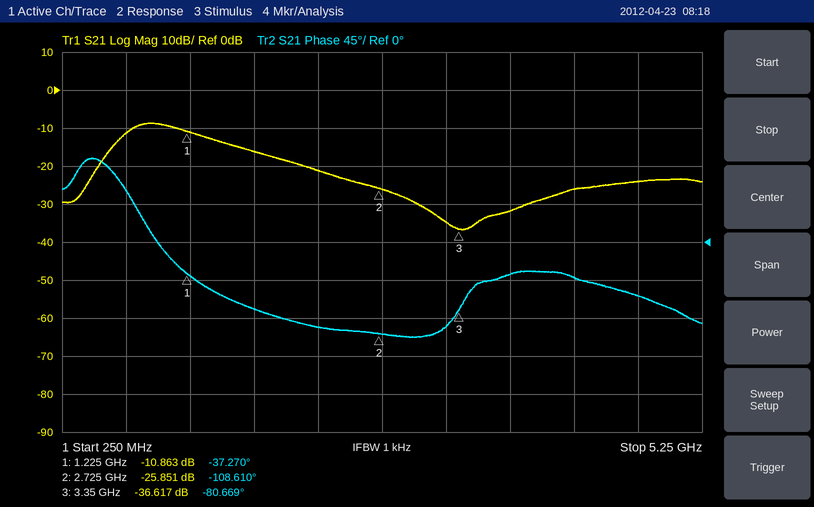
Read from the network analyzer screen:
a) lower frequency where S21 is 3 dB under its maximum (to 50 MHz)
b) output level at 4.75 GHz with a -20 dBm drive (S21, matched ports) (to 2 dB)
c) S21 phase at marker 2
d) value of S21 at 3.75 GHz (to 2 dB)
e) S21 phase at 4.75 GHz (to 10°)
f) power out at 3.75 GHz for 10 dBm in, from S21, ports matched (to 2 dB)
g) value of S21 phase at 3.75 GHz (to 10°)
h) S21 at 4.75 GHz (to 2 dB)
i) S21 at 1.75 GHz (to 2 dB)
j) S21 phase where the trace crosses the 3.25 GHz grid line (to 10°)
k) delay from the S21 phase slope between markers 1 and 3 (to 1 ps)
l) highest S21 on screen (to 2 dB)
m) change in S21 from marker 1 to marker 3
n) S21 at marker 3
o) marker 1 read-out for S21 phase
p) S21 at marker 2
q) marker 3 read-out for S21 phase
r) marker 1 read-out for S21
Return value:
750 MHz
-44 dBm
-108.610°
-32 dB
-60°
-22 dBm
-40°
-24 dB
-16 dB
-100°
57 ps
-8 dB
-25.754 dB
-36.617 dB
-37.270°
-25.851 dB
-80.669°
-10.863 dB
